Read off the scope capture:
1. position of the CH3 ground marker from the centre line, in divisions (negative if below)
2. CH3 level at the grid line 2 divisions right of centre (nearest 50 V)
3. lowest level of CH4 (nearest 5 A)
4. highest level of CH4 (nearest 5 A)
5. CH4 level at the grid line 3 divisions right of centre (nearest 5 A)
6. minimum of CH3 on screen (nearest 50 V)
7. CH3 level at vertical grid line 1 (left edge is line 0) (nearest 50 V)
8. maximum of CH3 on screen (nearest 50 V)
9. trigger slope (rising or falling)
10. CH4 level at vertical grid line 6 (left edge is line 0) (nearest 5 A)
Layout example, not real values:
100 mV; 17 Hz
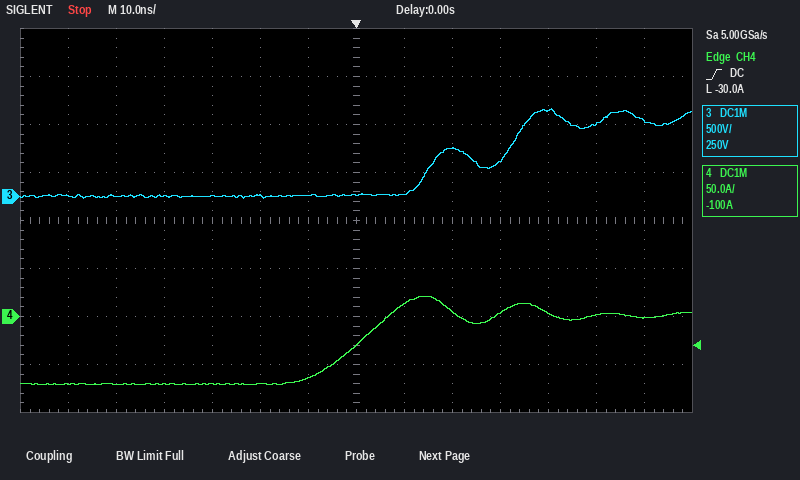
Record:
+0.5 div; 500 V; -70 A; 20 A; 5 A; 0 V; 0 V; 900 V; rising; -65 A
